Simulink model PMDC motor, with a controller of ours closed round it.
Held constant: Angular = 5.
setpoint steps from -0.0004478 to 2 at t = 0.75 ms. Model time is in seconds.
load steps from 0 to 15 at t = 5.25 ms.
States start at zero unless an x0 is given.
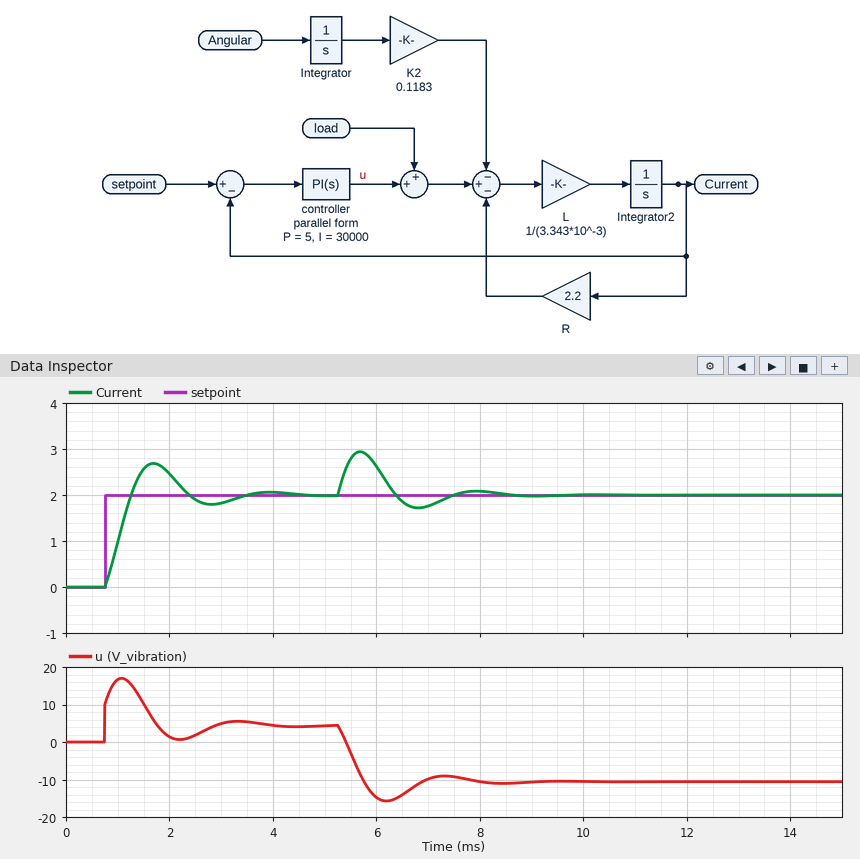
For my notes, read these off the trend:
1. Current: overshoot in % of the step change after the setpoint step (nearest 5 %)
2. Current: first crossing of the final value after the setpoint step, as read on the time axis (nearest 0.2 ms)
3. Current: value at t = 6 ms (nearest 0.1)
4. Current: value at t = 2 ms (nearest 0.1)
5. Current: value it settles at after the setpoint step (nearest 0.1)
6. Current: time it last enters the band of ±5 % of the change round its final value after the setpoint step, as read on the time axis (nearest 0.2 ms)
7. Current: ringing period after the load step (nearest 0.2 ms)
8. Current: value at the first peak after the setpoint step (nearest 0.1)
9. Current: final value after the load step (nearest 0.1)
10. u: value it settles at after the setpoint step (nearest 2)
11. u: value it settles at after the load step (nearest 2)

35 %
1.2 ms
2.6
2.5
2.0
3.2 ms
2.2 ms
2.7
2.0
4
-10
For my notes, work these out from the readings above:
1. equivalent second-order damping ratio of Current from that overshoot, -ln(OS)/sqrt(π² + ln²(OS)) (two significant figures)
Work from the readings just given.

0.32
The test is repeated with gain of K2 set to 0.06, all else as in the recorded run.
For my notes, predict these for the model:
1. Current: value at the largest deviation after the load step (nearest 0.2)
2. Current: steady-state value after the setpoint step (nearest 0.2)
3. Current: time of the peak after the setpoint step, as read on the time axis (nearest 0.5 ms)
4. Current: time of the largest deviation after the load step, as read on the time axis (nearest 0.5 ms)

3.0
2.0
1.5 ms
5.5 ms
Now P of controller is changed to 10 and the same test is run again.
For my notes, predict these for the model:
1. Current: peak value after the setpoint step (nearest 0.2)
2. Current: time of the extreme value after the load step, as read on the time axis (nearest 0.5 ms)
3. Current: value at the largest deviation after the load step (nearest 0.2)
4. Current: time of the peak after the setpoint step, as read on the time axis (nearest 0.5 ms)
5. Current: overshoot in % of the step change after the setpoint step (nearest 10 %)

2.4
5.5 ms
2.8
1.5 ms
20 %
